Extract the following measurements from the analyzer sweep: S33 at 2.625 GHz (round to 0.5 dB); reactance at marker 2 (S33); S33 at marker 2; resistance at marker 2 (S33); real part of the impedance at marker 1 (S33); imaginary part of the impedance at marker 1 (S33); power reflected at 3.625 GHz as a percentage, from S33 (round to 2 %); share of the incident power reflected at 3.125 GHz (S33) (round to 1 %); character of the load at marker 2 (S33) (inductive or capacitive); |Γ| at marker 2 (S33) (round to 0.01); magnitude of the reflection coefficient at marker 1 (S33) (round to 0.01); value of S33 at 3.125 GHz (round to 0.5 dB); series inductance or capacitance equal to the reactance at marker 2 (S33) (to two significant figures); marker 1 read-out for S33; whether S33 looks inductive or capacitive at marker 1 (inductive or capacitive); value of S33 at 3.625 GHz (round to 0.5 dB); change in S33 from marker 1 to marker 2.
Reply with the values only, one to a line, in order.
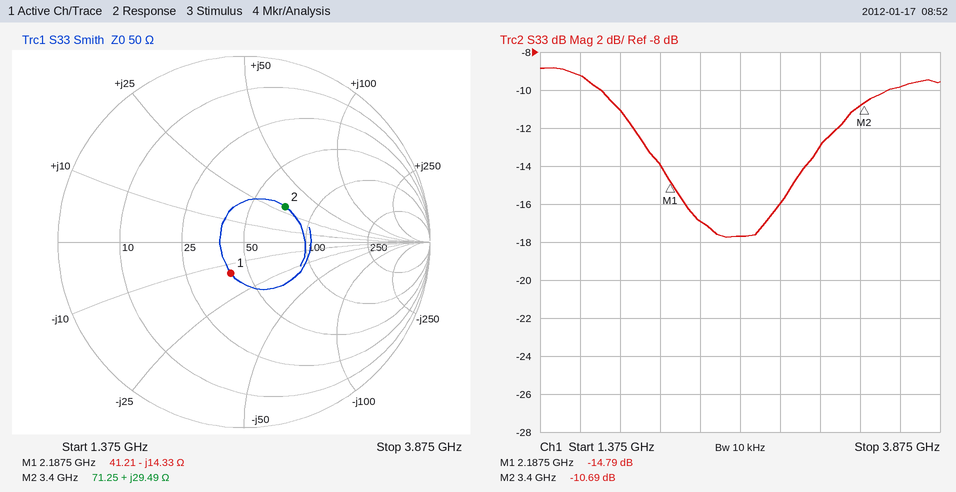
-17.5 dB
+29.49 Ω
-10.69 dB
71.25 Ω
41.21 Ω
-14.33 Ω
10 %
5 %
inductive
0.29
0.18
-13.0 dB
1.4 nH
-14.79 dB
capacitive
-10.0 dB
4.10 dB
